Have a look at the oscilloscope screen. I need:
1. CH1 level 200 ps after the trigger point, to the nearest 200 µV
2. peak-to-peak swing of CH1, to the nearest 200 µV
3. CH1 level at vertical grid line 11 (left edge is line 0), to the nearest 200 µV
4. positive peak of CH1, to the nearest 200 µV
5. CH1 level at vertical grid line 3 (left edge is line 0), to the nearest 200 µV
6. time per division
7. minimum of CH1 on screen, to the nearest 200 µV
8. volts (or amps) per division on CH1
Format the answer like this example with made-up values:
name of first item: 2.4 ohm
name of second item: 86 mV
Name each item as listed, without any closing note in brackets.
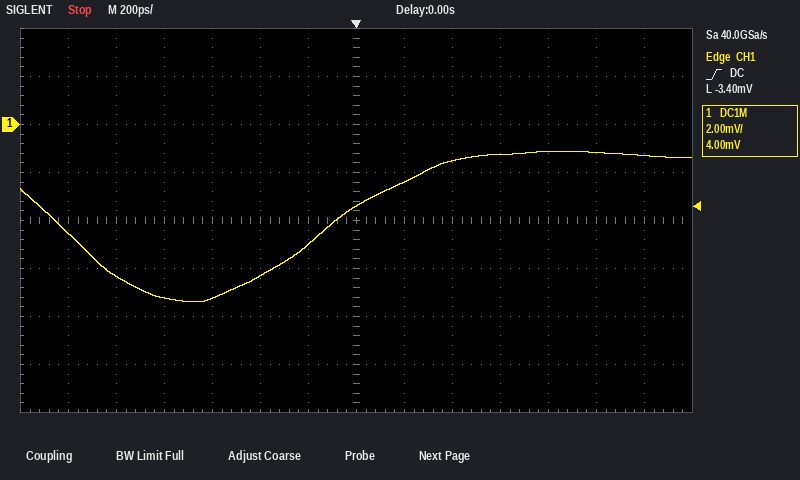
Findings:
CH1 level 200 ps after the trigger point, to the nearest 200 µV: -2.4 mV
peak-to-peak swing of CH1, to the nearest 200 µV: 6.2 mV
CH1 level at vertical grid line 11 (left edge is line 0), to the nearest 200 µV: -1.2 mV
positive peak of CH1, to the nearest 200 µV: -1.2 mV
CH1 level at vertical grid line 3 (left edge is line 0), to the nearest 200 µV: -7.2 mV
time per division: 200 ps
minimum of CH1 on screen, to the nearest 200 µV: -7.4 mV
volts (or amps) per division on CH1: 2 mV
